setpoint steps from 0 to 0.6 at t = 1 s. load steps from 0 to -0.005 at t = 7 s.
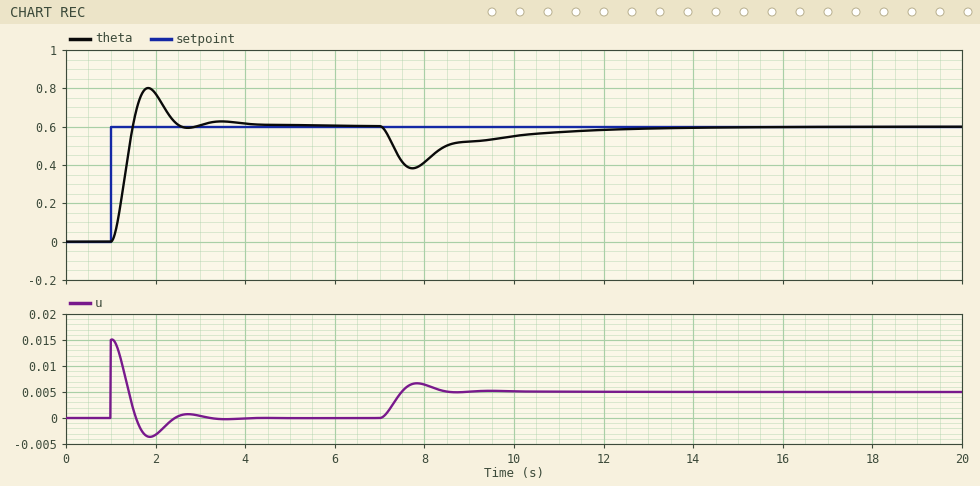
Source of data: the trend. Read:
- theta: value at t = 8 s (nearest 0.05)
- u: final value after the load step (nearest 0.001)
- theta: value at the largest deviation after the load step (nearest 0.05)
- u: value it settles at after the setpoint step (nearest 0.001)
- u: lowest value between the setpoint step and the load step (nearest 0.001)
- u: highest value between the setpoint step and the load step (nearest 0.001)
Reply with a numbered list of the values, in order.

1. 0.40
2. 0.005
3. 0.40
4. 0.000
5. -0.004
6. 0.015
